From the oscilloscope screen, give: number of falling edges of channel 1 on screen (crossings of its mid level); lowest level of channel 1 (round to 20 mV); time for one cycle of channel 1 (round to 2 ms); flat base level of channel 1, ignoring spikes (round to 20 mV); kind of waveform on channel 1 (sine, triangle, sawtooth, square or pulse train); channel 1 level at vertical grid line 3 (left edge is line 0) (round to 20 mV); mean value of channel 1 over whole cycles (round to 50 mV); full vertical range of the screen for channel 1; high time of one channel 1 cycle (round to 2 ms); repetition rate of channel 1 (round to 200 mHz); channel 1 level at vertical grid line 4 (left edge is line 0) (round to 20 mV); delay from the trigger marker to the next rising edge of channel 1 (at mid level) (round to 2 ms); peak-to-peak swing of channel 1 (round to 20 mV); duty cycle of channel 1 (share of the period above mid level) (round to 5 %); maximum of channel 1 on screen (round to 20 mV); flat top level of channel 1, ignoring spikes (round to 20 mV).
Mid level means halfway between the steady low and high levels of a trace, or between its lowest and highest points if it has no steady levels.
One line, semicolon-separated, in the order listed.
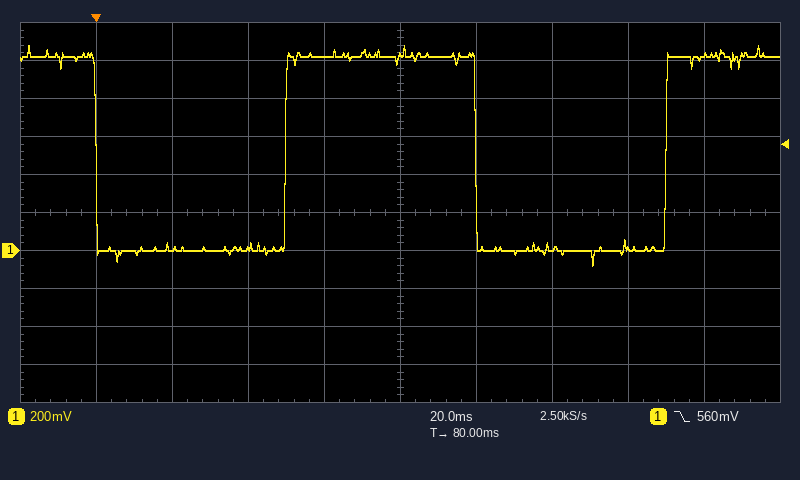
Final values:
2; -80 mV; 100 ms; 0 mV; square; 20 mV; 500 mV; 2 V; 50 ms; 10.0 Hz; 1.02 V; 50 ms; 1.16 V; 50 %; 1.08 V; 1.02 V
